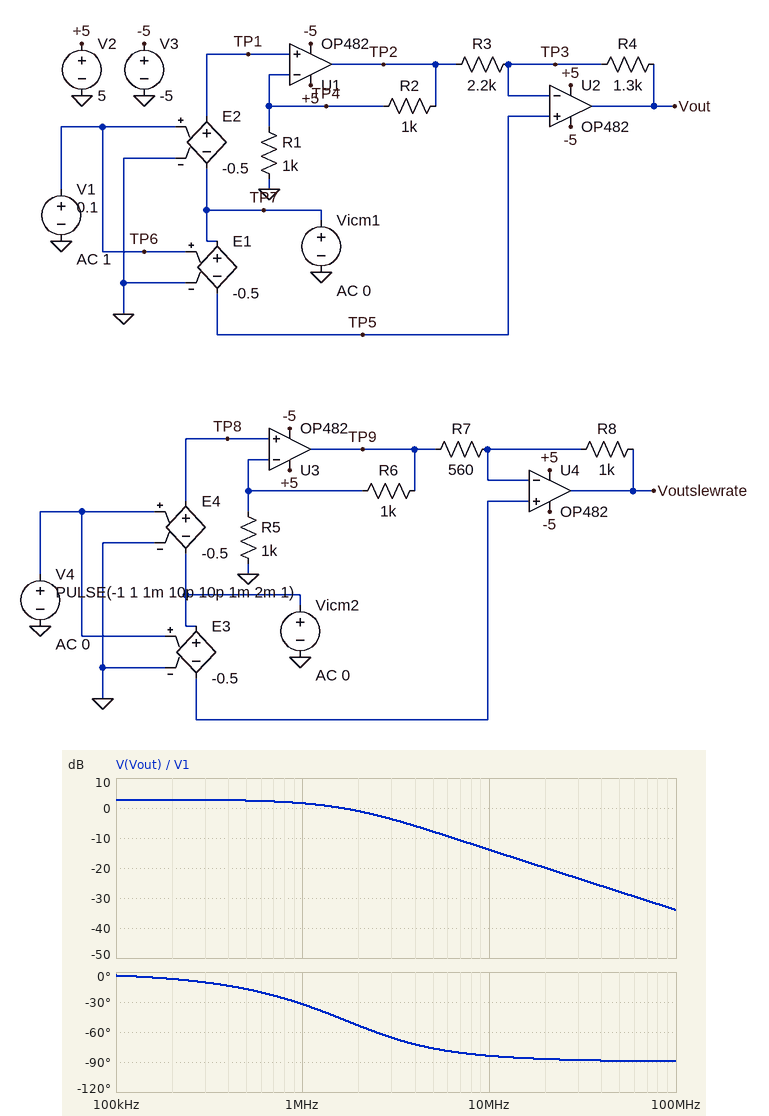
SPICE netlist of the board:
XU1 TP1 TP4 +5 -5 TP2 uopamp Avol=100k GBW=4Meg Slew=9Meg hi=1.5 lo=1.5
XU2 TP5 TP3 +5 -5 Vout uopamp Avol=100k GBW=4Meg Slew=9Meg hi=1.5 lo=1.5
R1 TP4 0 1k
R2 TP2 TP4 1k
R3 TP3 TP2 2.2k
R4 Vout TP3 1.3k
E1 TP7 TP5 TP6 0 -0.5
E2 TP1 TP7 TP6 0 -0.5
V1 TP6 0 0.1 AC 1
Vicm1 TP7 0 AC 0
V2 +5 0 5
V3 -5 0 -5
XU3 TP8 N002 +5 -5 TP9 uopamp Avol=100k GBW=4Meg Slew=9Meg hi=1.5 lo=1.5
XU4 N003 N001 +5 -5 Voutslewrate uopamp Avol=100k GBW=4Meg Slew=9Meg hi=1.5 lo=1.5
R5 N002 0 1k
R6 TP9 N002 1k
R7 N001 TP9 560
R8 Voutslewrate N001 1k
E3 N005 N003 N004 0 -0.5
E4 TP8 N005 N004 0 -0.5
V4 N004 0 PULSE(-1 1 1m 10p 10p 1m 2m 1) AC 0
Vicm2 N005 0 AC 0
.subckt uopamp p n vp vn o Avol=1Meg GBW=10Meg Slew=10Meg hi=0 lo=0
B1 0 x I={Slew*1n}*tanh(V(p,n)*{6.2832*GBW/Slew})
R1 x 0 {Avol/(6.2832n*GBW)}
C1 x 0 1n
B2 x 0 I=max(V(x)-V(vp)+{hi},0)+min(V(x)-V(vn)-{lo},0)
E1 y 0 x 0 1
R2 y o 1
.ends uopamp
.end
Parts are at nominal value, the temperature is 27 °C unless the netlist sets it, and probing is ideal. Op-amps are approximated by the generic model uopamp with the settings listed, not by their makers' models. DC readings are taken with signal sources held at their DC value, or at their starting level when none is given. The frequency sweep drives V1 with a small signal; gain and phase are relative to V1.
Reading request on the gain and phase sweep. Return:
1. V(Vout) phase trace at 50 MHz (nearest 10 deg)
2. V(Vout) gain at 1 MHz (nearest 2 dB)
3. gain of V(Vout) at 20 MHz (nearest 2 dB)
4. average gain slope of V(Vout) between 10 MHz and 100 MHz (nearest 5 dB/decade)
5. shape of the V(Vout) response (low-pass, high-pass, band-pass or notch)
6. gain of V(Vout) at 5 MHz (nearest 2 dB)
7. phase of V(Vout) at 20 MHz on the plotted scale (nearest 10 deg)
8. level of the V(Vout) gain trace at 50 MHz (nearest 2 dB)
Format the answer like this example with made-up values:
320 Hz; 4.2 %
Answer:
-90 deg; 2 dB; -20 dB; -20 dB/decade; low-pass; -8 dB; -90 deg; -28 dB
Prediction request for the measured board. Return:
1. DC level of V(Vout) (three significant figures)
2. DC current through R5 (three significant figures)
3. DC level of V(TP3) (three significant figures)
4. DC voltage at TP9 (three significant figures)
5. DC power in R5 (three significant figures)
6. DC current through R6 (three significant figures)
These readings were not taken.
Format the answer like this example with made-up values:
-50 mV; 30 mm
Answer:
139 mV; 500 µA; 50.0 mV; 1.00 V; 250 µW; 500 µA
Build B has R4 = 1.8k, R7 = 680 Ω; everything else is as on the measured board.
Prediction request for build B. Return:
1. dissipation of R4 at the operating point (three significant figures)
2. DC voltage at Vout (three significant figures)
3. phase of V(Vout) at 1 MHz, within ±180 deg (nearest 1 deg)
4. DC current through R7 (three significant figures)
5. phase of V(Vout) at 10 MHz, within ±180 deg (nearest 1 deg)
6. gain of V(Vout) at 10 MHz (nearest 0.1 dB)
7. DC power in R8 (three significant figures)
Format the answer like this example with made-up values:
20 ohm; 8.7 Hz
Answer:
8.37 µW; 173 mV; -36 deg; 2.21 mA; -87 deg; -13.8 dB; 4.87 mW
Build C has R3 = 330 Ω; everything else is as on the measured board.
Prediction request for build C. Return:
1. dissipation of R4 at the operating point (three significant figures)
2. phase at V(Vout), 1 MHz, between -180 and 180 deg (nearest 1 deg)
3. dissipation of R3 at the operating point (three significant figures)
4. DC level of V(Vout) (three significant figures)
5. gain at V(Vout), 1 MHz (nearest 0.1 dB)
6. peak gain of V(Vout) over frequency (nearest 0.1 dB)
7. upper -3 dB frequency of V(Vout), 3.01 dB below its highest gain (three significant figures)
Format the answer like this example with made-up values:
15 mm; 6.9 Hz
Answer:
269 µW; -67 deg; 68.2 µW; 641 mV; 11.3 dB; 16.1 dB; 724 kHz
